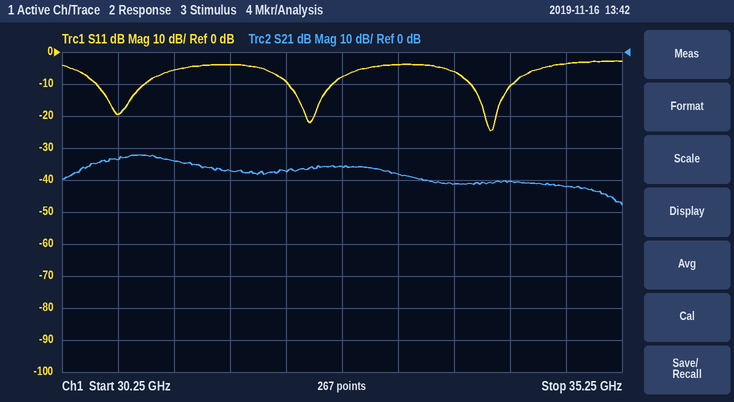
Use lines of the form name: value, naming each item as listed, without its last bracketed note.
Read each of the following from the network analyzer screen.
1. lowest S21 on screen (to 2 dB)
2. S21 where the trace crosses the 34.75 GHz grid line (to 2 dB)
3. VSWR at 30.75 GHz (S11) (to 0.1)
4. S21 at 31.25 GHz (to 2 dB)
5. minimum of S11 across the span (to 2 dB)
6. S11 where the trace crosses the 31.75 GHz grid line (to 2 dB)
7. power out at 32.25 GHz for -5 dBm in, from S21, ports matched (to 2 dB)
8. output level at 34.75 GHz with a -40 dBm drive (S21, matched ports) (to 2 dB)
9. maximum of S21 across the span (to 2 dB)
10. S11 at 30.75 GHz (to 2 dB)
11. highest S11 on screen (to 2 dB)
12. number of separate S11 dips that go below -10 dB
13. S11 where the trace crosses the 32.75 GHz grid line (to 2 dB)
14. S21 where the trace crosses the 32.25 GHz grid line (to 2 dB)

lowest S21 on screen: -48 dB
S21 where the trace crosses the 34.75 GHz grid line: -42 dB
VSWR at 30.75 GHz (S11): 1.2
S21 at 31.25 GHz: -34 dB
minimum of S11 across the span: -24 dB
S11 where the trace crosses the 31.75 GHz grid line: -4 dB
power out at 32.25 GHz for -5 dBm in, from S21, ports matched: -42 dBm
output level at 34.75 GHz with a -40 dBm drive (S21, matched ports): -82 dBm
maximum of S21 across the span: -32 dB
S11 at 30.75 GHz: -20 dB
highest S11 on screen: -2 dB
number of separate S11 dips that go below -10 dB: 3
S11 where the trace crosses the 32.75 GHz grid line: -8 dB
S21 where the trace crosses the 32.25 GHz grid line: -38 dB
